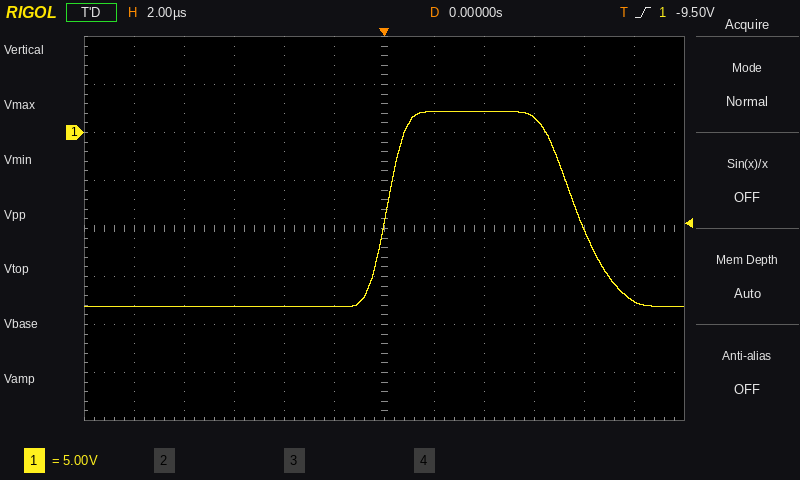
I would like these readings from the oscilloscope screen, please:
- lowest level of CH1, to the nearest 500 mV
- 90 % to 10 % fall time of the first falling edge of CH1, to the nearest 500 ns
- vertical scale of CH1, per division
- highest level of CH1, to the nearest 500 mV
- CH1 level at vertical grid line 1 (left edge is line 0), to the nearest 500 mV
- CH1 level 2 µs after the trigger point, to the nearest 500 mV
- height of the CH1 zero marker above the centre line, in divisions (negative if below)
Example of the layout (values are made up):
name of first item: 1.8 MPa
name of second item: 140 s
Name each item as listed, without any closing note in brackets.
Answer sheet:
lowest level of CH1, to the nearest 500 mV: -18.0 V
90 % to 10 % fall time of the first falling edge of CH1, to the nearest 500 ns: 3.0 µs
vertical scale of CH1, per division: 5 V
highest level of CH1, to the nearest 500 mV: 2.0 V
CH1 level at vertical grid line 1 (left edge is line 0), to the nearest 500 mV: -18.0 V
CH1 level 2 µs after the trigger point, to the nearest 500 mV: 2.0 V
height of the CH1 zero marker above the centre line, in divisions: +2.0 div
